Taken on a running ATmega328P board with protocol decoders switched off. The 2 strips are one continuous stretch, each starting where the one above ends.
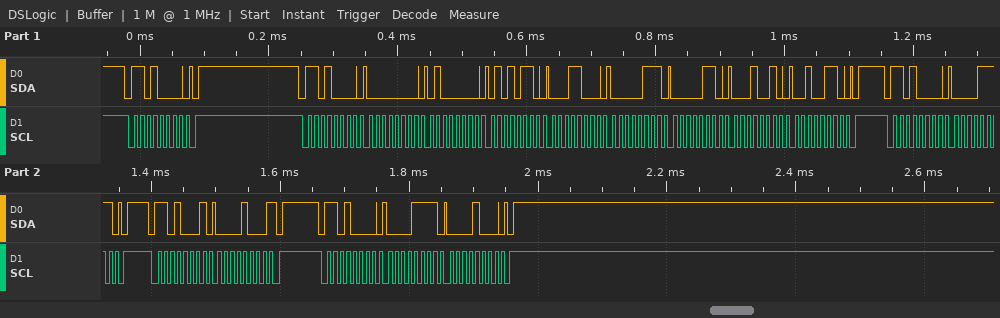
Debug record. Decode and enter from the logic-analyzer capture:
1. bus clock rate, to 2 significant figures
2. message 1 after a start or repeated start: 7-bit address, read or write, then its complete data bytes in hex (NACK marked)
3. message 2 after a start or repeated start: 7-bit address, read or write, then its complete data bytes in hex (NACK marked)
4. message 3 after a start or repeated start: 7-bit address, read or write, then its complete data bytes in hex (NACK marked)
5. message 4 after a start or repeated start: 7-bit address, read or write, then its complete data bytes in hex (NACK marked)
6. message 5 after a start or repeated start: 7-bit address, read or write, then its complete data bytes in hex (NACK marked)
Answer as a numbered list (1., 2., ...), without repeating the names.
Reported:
1. 100 kHz
2. 0x68 write
3. 0x68 write: 00 40 56 18 07 06 12 26
4. 0x68 write: 0F
5. 0x68 read: 08 NACK
6. 0x68 write: 0F 08
